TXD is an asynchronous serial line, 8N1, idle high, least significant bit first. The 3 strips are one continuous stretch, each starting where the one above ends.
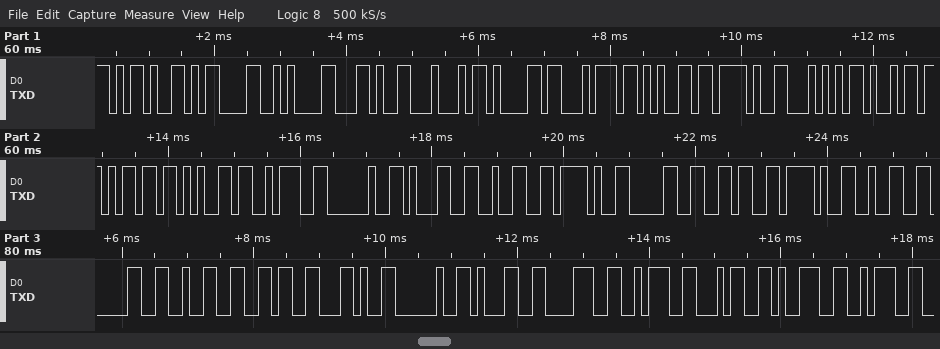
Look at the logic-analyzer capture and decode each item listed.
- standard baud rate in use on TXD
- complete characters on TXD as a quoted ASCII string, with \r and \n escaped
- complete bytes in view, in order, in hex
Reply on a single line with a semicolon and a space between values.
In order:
9600 baud; "-\r\n,Date/Time: 12/06/2026, 18:49:"; 2D 0D 0A 2C 44 61 74 65 2F 54 69 6D 65 3A 20 31 32 2F 30 36 2F 32 30 32 36 2C 20 31 38 3A 34 39 3A
